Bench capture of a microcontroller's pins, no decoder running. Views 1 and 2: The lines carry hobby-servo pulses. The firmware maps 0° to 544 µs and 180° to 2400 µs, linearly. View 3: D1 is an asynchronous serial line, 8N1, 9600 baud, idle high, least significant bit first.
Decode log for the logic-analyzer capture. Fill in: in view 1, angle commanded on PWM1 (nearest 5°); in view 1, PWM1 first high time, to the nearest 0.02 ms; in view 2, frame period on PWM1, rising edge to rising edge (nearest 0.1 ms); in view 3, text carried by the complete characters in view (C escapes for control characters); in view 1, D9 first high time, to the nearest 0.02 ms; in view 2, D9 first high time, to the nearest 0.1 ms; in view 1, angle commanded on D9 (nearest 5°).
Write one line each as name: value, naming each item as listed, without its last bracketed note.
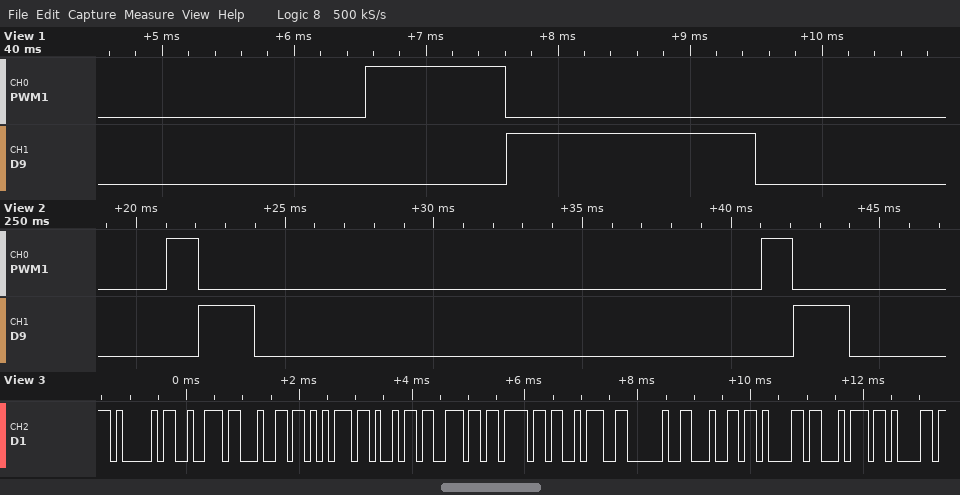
in view 1, angle commanded on PWM1: 50°
in view 1, PWM1 first high time, to the nearest 0.02 ms: 1.06 ms
in view 2, frame period on PWM1, rising edge to rising edge: 20.0 ms
in view 3, text carried by the complete characters in view: "Arduino: data"
in view 1, D9 first high time, to the nearest 0.02 ms: 1.88 ms
in view 2, D9 first high time, to the nearest 0.1 ms: 1.9 ms
in view 1, angle commanded on D9: 130°
